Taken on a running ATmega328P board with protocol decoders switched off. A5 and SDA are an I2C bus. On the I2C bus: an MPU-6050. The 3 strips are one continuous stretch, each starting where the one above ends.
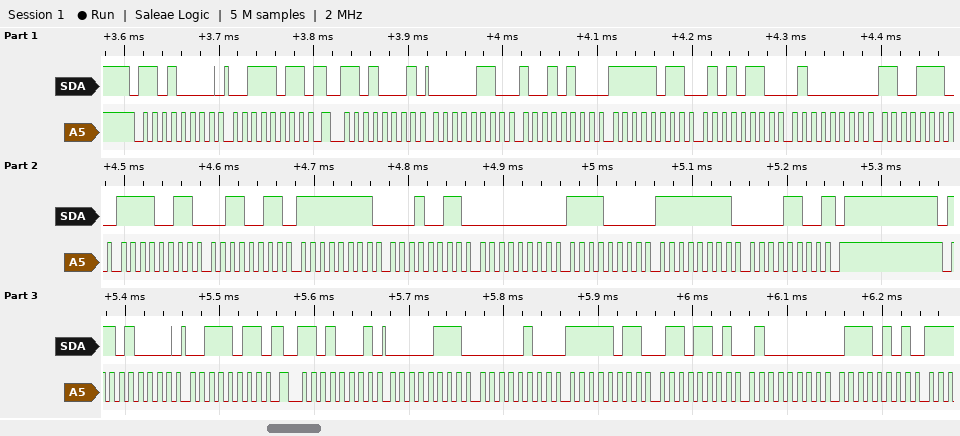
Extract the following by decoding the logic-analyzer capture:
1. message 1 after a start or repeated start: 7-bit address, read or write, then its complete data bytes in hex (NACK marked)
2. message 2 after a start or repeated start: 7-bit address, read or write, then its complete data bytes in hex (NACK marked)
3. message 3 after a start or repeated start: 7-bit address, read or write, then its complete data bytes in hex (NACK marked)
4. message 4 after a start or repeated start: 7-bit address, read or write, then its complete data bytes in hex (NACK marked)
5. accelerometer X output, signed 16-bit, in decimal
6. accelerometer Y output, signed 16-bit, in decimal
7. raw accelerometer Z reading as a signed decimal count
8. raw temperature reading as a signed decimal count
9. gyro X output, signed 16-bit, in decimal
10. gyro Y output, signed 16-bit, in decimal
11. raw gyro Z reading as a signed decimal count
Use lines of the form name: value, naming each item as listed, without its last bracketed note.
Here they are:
message 1 after a start or repeated start: 7-bit address, read or write, then its complete data bytes in hex: 0x68 write: 3B
message 2 after a start or repeated start: 7-bit address, read or write, then its complete data bytes in hex: 0x68 read: 06 94 FB 56 40 CE F3 33 FF 13 00 F0 FF 0C NACK
message 3 after a start or repeated start: 7-bit address, read or write, then its complete data bytes in hex: 0x68 write: 3B
message 4 after a start or repeated start: 7-bit address, read or write, then its complete data bytes in hex: 0x68 read: 07 04 FB 6D 40 75
accelerometer X output, signed 16-bit, in decimal: 1684
accelerometer Y output, signed 16-bit, in decimal: -1194
raw accelerometer Z reading as a signed decimal count: 16590
raw temperature reading as a signed decimal count: -3277
gyro X output, signed 16-bit, in decimal: -237
gyro Y output, signed 16-bit, in decimal: 240
raw gyro Z reading as a signed decimal count: -244
